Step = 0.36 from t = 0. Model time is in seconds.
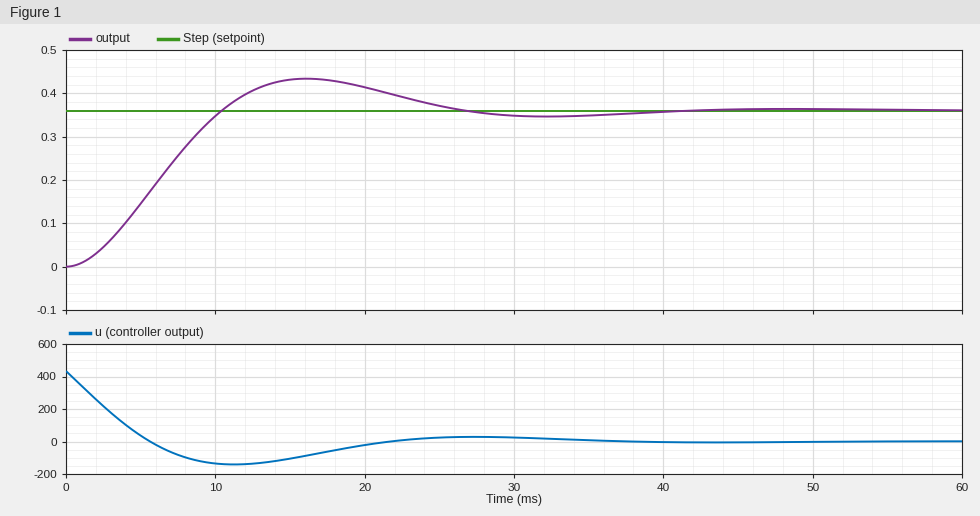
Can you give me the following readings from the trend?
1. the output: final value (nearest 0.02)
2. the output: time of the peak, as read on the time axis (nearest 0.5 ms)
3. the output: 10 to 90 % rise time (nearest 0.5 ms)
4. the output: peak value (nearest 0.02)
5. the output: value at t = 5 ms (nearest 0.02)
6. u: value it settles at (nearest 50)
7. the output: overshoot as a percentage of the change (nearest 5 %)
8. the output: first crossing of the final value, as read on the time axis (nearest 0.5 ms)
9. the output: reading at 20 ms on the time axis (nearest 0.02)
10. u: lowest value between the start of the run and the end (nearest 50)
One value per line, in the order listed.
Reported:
0.36
16.0 ms
7.0 ms
0.44
0.14
0
20 %
10.5 ms
0.42
-150
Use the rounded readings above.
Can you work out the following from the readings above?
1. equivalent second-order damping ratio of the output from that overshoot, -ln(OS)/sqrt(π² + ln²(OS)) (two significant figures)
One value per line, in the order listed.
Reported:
0.46
